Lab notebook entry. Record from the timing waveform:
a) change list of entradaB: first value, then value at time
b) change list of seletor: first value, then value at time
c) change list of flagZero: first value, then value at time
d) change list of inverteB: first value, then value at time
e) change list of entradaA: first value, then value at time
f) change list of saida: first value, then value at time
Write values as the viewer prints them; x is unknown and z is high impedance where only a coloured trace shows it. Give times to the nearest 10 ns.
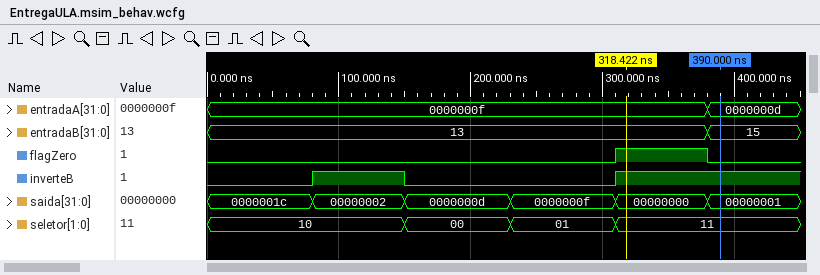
13, 15 at 380 ns
10, 00 at 150 ns, 01 at 230 ns, 11 at 310 ns
0, 1 at 310 ns, 0 at 380 ns
0, 1 at 80 ns, 0 at 150 ns, 1 at 310 ns
0000000f, 0000000d at 380 ns
0000001c, 00000002 at 80 ns, 0000000d at 150 ns, 0000000f at 230 ns, 00000000 at 310 ns, 00000001 at 380 ns
